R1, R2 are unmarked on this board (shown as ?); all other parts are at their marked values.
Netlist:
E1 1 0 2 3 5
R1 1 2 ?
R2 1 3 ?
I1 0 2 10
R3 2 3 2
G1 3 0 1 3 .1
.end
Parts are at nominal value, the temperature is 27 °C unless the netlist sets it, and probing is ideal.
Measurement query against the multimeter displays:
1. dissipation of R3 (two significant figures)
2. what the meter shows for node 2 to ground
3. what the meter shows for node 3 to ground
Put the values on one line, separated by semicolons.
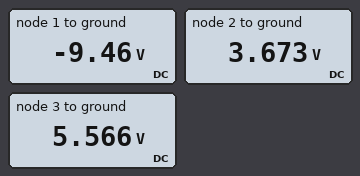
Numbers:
1.8 W; 3.673 V; 5.566 V
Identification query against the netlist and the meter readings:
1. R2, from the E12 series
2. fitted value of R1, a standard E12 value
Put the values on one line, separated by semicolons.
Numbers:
27 Ω; 1.2 Ω
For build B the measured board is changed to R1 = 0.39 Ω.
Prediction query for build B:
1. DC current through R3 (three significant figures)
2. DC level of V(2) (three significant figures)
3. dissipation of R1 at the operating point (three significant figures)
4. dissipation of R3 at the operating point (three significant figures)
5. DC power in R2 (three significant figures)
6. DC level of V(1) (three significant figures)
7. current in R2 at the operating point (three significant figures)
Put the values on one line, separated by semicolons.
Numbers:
289 mA; 1.12 V; 41.3 W; 167 mW; 781 mW; -2.89 V; 170 mA
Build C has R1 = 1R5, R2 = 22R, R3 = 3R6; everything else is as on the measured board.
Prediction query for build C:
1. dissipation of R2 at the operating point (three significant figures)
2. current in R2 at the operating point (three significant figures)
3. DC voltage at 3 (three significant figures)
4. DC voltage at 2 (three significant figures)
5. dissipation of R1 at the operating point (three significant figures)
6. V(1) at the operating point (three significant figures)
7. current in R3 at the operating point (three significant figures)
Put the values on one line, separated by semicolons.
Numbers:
19.6 W; 945 mA; 378 mV; -3.70 V; 186 W; -20.4 V; 1.13 A
